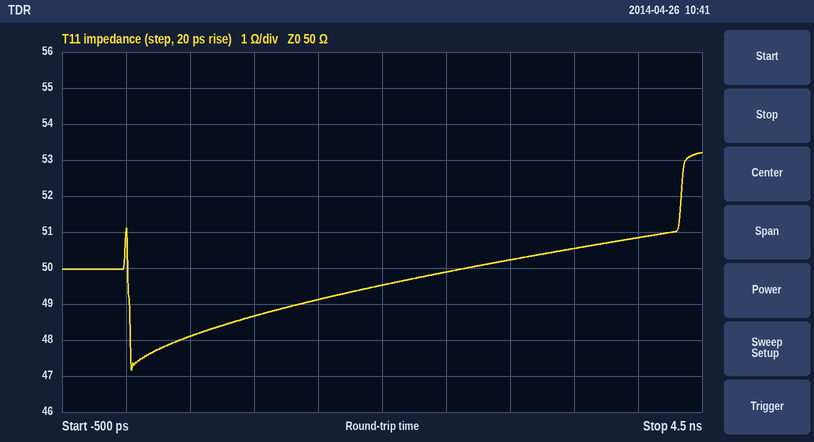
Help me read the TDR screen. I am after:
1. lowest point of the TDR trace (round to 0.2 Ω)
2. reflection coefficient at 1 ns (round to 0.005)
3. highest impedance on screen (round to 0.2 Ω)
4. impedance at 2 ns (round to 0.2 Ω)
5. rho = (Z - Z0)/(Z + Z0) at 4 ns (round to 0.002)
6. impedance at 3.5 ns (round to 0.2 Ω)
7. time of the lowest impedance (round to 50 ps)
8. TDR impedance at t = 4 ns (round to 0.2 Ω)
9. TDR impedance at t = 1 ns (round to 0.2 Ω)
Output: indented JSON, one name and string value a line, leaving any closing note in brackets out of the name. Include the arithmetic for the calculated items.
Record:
{
  "lowest point of the TDR trace": "47.2 Ω",
  "reflection coefficient at 1 ns": "(48.6 − 50)/(48.6 + 50) ≈ -0.0142, so -0.015 to the nearest 0.005",
  "highest impedance on screen": "53.2 Ω",
  "impedance at 2 ns": "49.6 Ω",
  "rho = (Z - Z0)/(Z + Z0) at 4 ns": "(50.8 − 50)/(50.8 + 50) ≈ +0.008",
  "impedance at 3.5 ns": "50.6 Ω",
  "time of the lowest impedance": "50 ps",
  "TDR impedance at t = 4 ns": "50.8 Ω",
  "TDR impedance at t = 1 ns": "48.6 Ω"
}
